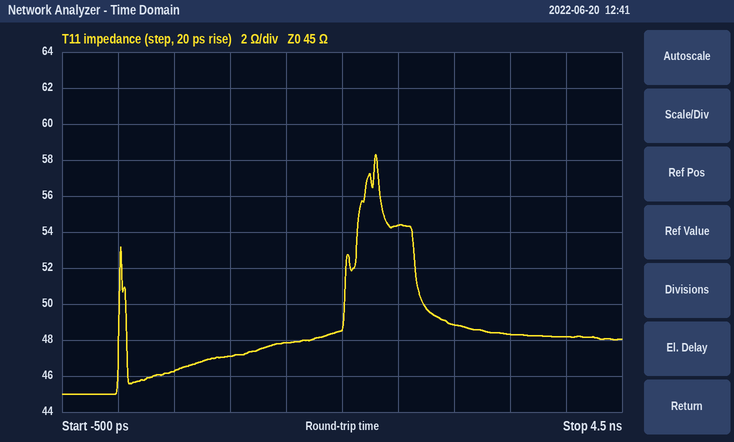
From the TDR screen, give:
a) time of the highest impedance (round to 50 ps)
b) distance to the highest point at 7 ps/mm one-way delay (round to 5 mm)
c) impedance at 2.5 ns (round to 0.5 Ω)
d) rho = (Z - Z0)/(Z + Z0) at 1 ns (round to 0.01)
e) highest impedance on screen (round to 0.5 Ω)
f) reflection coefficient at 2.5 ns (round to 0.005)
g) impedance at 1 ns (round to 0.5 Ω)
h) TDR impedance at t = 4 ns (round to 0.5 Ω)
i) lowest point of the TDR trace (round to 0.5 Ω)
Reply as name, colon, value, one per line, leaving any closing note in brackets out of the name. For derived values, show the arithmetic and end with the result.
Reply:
time of the highest impedance: 2.30 ns
distance to the highest point at 7 ps/mm one-way delay: 2.30 ns / 2 / 7 ps/mm ≈ 164 mm, so 165 mm to the nearest 5 mm
impedance at 2.5 ns: 54.5 Ω
rho = (Z - Z0)/(Z + Z0) at 1 ns: (47 − 45)/(47 + 45) ≈ +0.02
highest impedance on screen: 58.5 Ω
reflection coefficient at 2.5 ns: (54.5 − 45)/(54.5 + 45) ≈ +0.095
impedance at 1 ns: 47.0 Ω
TDR impedance at t = 4 ns: 48.0 Ω
lowest point of the TDR trace: 45.0 Ω
